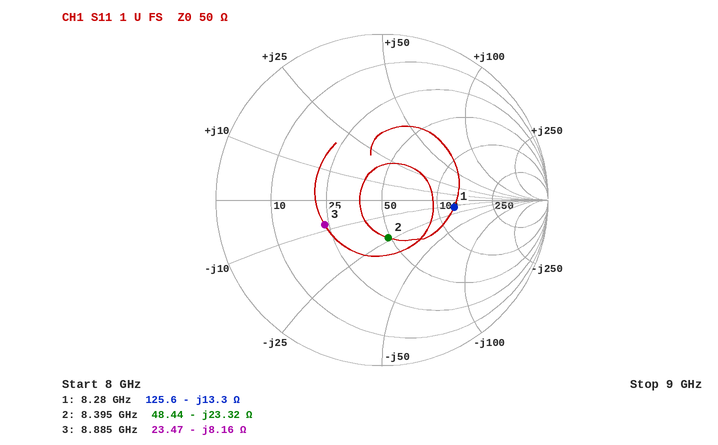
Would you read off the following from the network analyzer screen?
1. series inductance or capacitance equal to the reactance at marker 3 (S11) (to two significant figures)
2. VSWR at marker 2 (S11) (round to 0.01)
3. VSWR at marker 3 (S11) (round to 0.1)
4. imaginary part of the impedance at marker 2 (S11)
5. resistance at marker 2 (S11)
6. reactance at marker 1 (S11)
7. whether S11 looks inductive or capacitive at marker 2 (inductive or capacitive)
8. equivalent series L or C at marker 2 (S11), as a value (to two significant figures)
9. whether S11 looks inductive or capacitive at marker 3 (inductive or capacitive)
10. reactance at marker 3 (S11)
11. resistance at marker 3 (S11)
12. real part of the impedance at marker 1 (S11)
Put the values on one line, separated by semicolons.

2.2 pF; 1.60; 2.2; -23.32 Ω; 48.44 Ω; -13.3 Ω; capacitive; 810 fF; capacitive; -8.16 Ω; 23.47 Ω; 125.6 Ω
